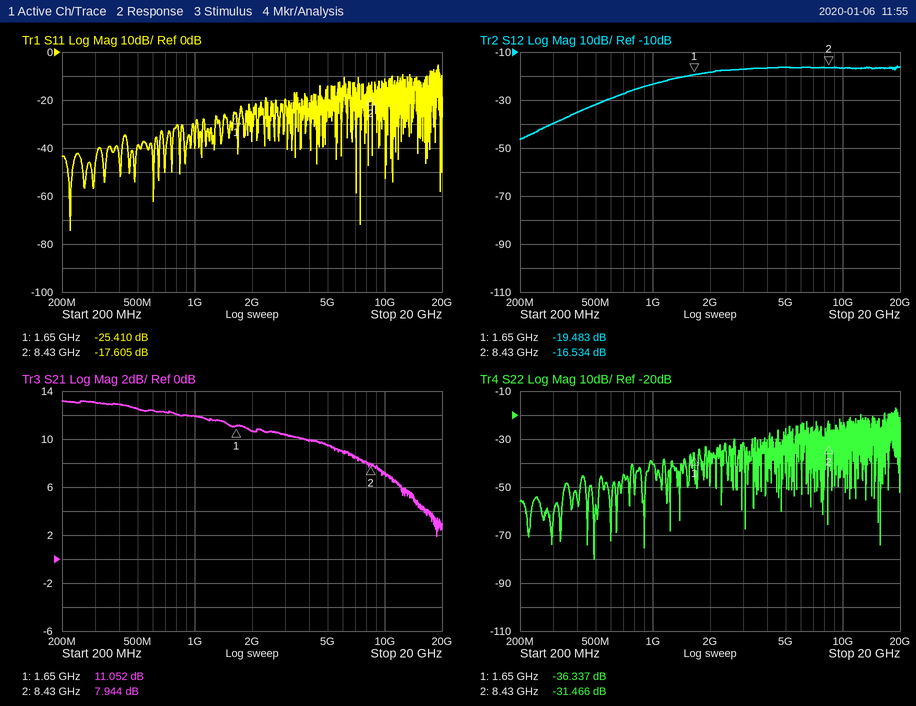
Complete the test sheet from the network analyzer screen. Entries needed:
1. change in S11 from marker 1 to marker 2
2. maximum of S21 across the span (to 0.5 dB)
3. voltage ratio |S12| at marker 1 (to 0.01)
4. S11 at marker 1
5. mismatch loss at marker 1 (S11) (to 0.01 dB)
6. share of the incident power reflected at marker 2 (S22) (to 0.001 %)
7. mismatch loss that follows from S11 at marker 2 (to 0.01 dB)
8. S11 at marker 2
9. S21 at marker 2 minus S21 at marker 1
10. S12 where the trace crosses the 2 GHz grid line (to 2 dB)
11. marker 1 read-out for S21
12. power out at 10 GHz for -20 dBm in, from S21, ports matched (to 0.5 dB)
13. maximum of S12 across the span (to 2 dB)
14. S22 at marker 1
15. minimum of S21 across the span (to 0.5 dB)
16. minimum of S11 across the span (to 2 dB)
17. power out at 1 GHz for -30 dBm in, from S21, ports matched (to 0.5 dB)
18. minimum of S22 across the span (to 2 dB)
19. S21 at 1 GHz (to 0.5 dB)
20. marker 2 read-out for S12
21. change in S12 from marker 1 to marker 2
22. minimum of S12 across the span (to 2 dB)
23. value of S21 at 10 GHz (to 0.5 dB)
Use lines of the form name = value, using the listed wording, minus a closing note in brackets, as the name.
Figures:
change in S11 from marker 1 to marker 2 = 7.805 dB
maximum of S21 across the span = 13.0 dB
voltage ratio |S12| at marker 1 = 0.11
S11 at marker 1 = -25.410 dB
mismatch loss at marker 1 (S11) = 0.01 dB
share of the incident power reflected at marker 2 (S22) = 0.071 %
mismatch loss that follows from S11 at marker 2 = 0.08 dB
S11 at marker 2 = -17.605 dB
S21 at marker 2 minus S21 at marker 1 = -3.108 dB
S12 where the trace crosses the 2 GHz grid line = -18 dB
marker 1 read-out for S21 = 11.052 dB
power out at 10 GHz for -20 dBm in, from S21, ports matched = -13.0 dBm
maximum of S12 across the span = -16 dB
S22 at marker 1 = -36.337 dB
minimum of S21 across the span = 2.0 dB
minimum of S11 across the span = -74 dB
power out at 1 GHz for -30 dBm in, from S21, ports matched = -18.0 dBm
minimum of S22 across the span = -80 dB
S21 at 1 GHz = 12.0 dB
marker 2 read-out for S12 = -16.534 dB
change in S12 from marker 1 to marker 2 = 2.949 dB
minimum of S12 across the span = -46 dB
value of S21 at 10 GHz = 7.0 dB
